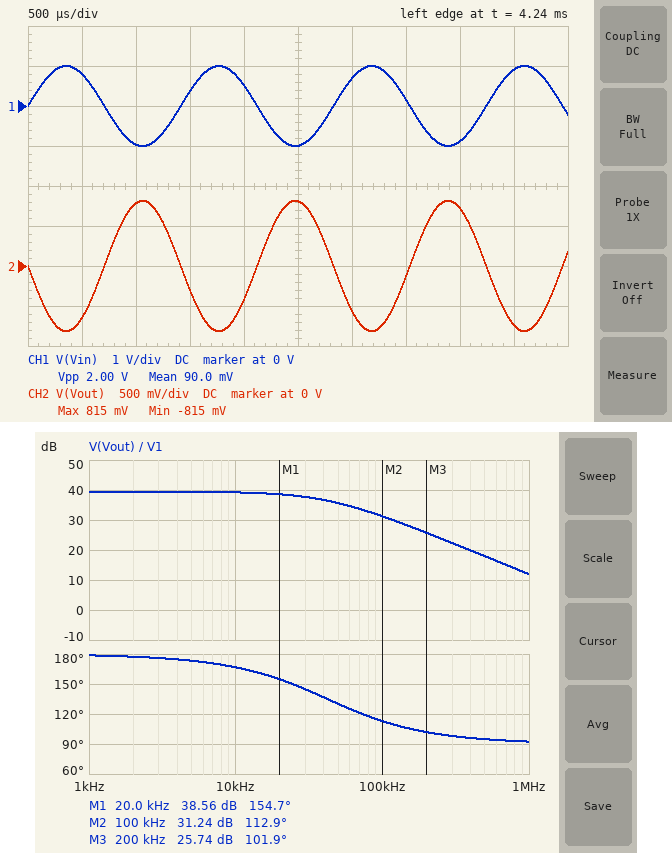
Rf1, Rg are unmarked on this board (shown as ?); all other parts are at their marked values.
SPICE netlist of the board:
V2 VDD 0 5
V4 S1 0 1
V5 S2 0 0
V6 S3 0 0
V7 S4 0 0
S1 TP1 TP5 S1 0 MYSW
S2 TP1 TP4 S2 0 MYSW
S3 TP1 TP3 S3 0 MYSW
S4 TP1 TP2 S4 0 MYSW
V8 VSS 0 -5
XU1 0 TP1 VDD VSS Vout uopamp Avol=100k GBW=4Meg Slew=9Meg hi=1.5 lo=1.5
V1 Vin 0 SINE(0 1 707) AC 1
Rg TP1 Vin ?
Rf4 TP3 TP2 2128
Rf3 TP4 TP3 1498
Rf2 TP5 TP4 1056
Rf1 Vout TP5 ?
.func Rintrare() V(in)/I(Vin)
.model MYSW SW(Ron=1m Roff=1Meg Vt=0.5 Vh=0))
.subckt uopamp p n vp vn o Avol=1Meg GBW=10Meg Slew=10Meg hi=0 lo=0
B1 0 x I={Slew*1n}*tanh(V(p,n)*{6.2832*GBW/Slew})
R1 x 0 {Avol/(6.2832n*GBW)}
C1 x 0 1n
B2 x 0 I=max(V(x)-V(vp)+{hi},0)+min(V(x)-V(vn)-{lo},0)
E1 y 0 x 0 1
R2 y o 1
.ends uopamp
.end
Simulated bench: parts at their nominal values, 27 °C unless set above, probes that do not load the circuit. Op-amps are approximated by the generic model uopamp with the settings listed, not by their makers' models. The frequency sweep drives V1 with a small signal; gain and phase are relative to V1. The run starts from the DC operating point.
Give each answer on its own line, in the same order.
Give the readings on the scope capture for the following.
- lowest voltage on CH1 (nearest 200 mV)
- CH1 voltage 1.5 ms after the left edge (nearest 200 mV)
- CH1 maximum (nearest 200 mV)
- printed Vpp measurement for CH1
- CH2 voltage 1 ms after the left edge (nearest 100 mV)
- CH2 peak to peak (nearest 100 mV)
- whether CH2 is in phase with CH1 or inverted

-1.0 V
400 mV
1.0 V
2.00 V
800 mV
1.6 V
inverted
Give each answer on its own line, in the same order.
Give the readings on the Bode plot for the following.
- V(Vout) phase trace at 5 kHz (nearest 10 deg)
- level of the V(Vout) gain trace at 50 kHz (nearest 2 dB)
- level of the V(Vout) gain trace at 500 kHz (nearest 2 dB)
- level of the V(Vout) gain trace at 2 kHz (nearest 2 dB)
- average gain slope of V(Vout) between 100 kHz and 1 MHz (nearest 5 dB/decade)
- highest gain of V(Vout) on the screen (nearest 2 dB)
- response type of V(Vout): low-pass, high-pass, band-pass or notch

170 deg
36 dB
18 dB
40 dB
-20 dB/decade
40 dB
low-pass
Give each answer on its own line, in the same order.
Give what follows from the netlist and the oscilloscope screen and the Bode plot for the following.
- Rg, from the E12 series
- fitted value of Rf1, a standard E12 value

2.7 kΩ
2.2 kΩ
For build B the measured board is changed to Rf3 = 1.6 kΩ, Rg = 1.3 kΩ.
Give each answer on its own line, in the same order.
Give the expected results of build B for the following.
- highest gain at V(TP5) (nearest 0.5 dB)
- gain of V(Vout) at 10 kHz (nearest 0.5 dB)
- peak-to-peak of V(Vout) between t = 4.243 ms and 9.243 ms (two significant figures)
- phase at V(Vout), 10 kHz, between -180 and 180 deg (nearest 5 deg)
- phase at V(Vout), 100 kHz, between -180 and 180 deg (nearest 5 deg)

45.5 dB
45.0 dB
3.4 V
155 deg
100 deg
